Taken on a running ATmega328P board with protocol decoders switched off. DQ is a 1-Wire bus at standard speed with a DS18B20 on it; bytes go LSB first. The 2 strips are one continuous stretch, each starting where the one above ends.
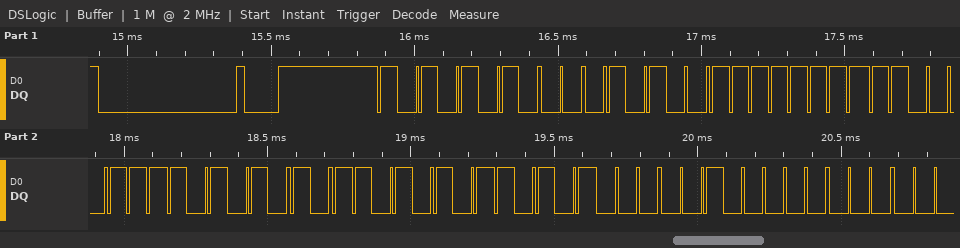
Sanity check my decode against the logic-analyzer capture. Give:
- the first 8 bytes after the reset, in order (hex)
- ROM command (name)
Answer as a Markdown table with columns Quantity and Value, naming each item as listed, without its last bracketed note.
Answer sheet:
| Quantity | Value |
|---|---|
| the first 8 bytes after the reset, in order | 55 28 FF E3 55 AB 15 04 |
| ROM command | Match ROM |
